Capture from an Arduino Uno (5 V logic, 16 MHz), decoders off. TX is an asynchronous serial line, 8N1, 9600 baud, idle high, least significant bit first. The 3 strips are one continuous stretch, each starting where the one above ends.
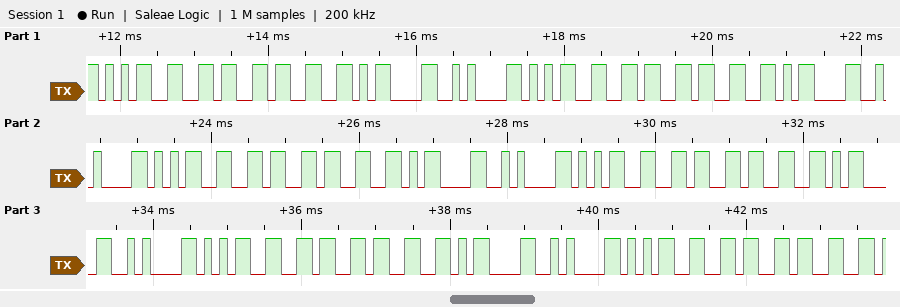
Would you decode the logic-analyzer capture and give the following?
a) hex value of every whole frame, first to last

35 36 33 0D 0A 35 36 33 0D 0A 35 36 33 0D 0A 35 36 33 0D 0A 35 36 33 0D 0A 35 36 33
